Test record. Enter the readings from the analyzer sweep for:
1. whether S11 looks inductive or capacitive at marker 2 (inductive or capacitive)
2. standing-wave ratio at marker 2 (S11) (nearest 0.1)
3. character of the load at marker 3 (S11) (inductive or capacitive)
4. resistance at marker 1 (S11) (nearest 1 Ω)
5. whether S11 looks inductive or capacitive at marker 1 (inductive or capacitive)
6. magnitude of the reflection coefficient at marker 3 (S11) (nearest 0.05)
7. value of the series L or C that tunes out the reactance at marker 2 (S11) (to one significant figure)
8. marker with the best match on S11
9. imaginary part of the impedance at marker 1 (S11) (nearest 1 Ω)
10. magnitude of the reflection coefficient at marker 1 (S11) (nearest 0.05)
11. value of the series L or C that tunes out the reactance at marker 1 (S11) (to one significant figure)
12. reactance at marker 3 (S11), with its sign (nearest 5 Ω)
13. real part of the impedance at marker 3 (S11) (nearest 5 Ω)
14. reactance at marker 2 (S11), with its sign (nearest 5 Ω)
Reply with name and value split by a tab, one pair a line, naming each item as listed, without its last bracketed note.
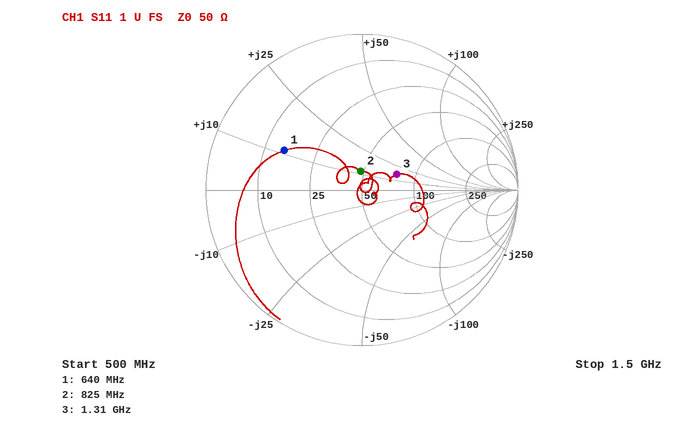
whether S11 looks inductive or capacitive at marker 2	inductive
standing-wave ratio at marker 2 (S11)	1.3
character of the load at marker 3 (S11)	inductive
resistance at marker 1 (S11)	15 Ω
whether S11 looks inductive or capacitive at marker 1	inductive
magnitude of the reflection coefficient at marker 3 (S11)	0.25
value of the series L or C that tunes out the reactance at marker 2 (S11)	20 pF
marker with the best match on S11	marker 2
imaginary part of the impedance at marker 1 (S11)	+11 Ω
magnitude of the reflection coefficient at marker 1 (S11)	0.55
value of the series L or C that tunes out the reactance at marker 1 (S11)	20 pF
reactance at marker 3 (S11), with its sign	+15 Ω
real part of the impedance at marker 3 (S11)	75 Ω
reactance at marker 2 (S11), with its sign	+10 Ω
